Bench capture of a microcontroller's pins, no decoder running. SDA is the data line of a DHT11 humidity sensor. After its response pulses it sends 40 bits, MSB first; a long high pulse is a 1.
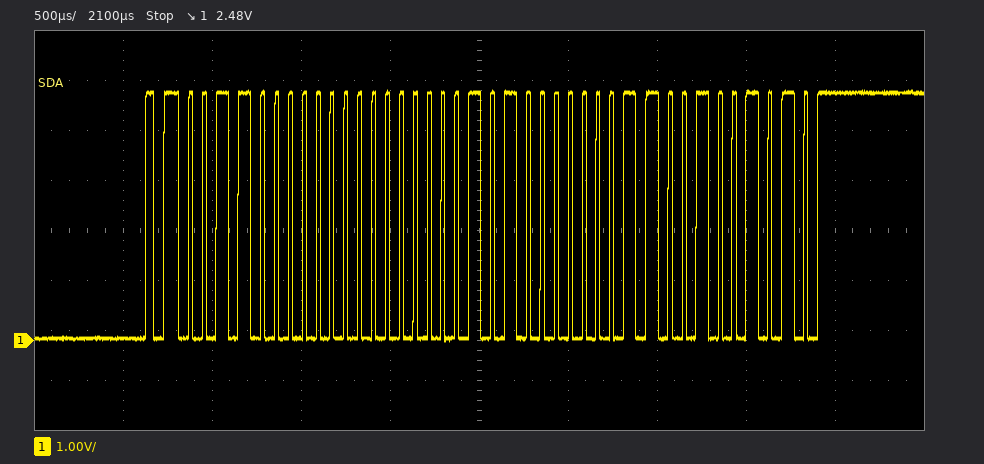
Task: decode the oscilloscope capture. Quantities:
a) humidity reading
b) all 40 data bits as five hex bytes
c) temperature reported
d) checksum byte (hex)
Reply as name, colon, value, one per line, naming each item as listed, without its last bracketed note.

humidity reading: 48 %
all 40 data bits as five hex bytes: 30 00 14 06 4A
temperature reported: 20.6 °C
checksum byte: 0x4A
